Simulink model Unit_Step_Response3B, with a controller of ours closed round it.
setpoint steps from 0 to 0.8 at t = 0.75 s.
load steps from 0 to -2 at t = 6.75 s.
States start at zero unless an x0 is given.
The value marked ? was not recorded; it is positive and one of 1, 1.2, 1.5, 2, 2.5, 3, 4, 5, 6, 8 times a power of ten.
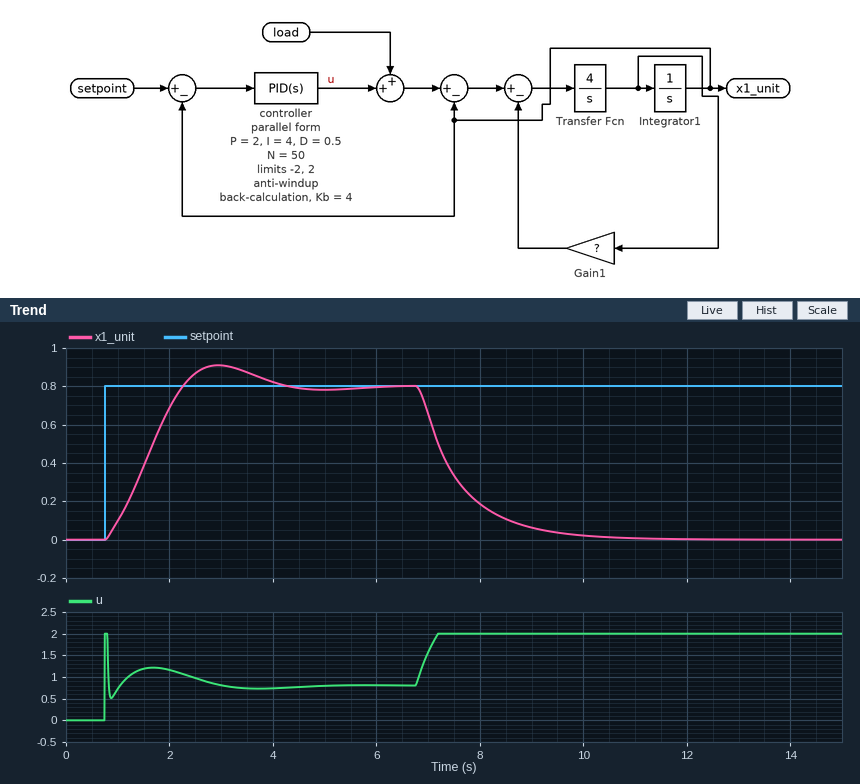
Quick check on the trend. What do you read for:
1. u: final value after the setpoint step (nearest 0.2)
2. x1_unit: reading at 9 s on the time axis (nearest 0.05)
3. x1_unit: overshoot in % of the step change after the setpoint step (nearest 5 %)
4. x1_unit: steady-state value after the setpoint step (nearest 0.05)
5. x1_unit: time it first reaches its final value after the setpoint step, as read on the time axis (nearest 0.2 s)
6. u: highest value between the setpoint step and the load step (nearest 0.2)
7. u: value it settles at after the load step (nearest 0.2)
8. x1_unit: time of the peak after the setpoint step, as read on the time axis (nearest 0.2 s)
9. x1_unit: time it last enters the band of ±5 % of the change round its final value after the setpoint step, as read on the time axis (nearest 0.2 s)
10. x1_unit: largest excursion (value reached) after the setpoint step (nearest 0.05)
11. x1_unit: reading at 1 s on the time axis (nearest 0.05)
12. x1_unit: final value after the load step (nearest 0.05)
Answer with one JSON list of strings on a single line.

["0.8", "0.05", "15 %", "0.80", "2.2 s", "2.0", "2.0", "3.0 s", "3.8 s", "0.90", "0.10", "0.00"]
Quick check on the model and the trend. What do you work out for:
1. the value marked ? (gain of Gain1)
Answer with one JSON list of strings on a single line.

["1.2"]
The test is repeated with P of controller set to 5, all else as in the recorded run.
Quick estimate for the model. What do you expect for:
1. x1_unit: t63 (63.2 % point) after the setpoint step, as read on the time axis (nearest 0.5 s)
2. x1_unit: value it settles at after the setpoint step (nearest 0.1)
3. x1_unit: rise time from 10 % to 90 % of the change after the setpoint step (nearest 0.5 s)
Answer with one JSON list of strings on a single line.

["1.5 s", "0.8", "2.0 s"]
